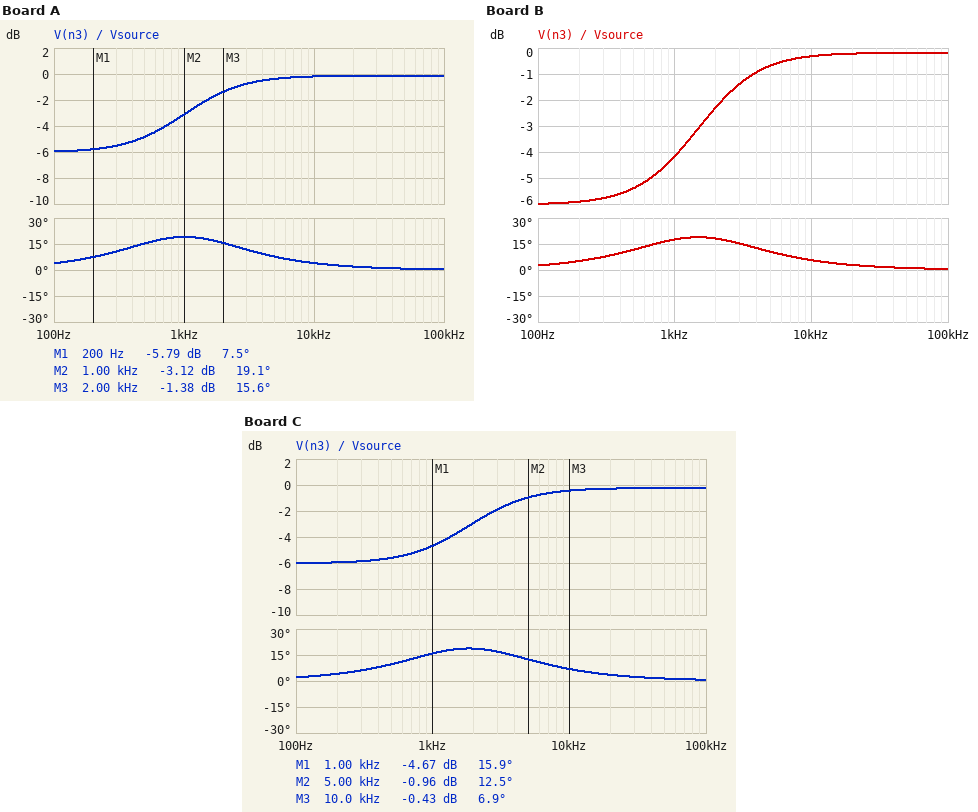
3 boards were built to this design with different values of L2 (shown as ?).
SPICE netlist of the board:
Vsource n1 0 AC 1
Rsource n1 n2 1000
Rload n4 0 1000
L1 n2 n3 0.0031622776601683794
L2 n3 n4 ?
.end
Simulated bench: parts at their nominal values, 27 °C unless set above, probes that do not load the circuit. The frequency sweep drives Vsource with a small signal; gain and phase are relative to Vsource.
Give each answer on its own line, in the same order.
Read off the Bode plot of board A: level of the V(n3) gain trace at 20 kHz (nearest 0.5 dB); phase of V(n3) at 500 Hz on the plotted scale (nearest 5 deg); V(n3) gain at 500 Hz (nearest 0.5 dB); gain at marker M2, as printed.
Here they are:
0 dB
15 deg
-5.0 dB
-3.12 dB
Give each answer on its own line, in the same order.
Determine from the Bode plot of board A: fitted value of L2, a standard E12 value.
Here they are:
220 mH
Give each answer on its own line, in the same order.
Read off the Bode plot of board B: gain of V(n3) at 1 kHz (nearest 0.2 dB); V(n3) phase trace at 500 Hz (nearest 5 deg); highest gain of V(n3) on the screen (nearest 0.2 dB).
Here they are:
-4.2 dB
10 deg
-0.2 dB
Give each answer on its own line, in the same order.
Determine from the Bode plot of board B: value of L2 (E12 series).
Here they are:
150 mH
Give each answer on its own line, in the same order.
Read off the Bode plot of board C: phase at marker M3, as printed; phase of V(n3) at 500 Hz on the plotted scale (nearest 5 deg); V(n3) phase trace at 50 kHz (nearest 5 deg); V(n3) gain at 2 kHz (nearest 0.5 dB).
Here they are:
6.9 deg
10 deg
0 deg
-3.0 dB
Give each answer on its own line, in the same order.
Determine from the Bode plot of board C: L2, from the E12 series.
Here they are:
120 mH
